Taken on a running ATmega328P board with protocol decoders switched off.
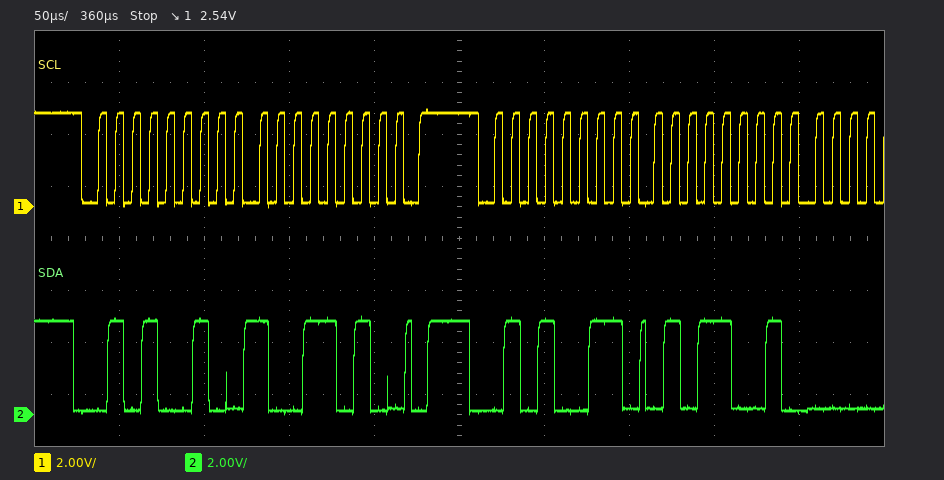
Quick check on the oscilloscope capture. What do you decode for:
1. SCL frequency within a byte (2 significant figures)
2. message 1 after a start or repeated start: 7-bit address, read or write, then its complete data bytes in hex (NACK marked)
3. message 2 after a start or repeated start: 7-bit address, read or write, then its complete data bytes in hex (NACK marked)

100 kHz
0x29 write: 9A
0x29 read: 59
